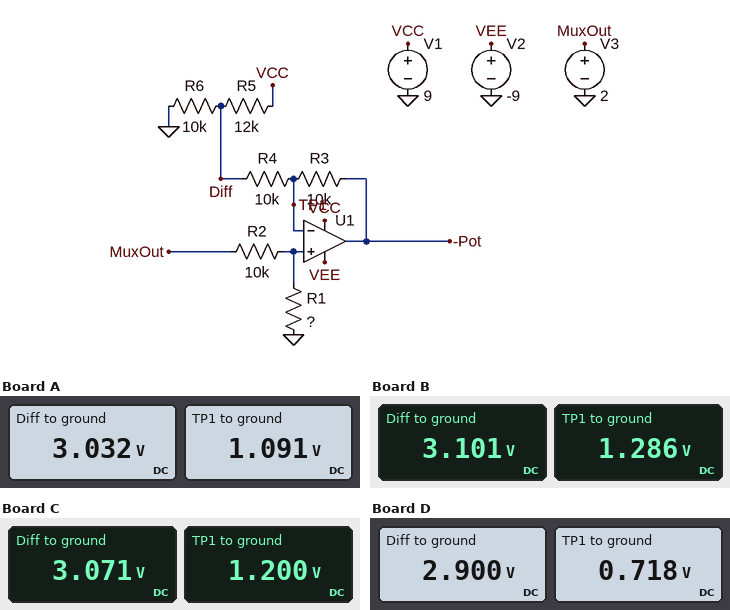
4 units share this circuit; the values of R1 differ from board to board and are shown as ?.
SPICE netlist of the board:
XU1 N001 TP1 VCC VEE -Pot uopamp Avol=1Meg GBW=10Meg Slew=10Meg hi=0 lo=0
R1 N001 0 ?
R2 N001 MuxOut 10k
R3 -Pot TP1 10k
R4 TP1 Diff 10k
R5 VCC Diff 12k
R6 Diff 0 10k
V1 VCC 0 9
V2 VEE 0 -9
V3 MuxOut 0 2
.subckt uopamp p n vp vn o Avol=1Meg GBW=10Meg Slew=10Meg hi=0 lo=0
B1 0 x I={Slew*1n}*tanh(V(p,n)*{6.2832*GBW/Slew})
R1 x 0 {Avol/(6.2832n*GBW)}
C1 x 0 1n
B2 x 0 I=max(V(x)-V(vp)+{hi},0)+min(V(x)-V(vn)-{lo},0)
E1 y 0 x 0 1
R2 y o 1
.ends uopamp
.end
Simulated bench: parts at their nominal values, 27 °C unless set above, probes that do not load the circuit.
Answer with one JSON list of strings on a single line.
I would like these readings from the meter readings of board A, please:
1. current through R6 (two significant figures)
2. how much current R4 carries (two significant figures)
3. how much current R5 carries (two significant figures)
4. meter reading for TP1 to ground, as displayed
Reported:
["300 µA", "190 µA", "500 µA", "1.091 V"]
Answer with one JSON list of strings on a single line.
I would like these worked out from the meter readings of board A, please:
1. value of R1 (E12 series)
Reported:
["12 kΩ"]
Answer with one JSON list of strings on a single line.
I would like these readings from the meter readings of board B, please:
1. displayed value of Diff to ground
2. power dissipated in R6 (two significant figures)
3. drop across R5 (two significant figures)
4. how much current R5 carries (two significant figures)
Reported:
["3.101 V", "960 µW", "5.9 V", "490 µA"]
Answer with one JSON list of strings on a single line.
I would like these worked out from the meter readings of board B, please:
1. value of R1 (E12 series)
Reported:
["18 kΩ"]
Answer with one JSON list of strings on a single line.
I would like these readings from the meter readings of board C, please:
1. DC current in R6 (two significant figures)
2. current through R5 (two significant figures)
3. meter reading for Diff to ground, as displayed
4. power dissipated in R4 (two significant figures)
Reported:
["310 µA", "490 µA", "3.071 V", "350 µW"]
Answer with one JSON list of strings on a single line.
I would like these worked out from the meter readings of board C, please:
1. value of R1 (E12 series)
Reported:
["15 kΩ"]
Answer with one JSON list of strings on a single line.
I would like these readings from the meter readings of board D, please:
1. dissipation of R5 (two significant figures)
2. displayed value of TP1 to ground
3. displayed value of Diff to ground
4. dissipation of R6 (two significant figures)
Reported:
["3.1 mW", "0.718 V", "2.900 V", "840 µW"]
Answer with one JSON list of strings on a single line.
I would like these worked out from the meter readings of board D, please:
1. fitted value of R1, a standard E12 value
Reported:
["5.6 kΩ"]
